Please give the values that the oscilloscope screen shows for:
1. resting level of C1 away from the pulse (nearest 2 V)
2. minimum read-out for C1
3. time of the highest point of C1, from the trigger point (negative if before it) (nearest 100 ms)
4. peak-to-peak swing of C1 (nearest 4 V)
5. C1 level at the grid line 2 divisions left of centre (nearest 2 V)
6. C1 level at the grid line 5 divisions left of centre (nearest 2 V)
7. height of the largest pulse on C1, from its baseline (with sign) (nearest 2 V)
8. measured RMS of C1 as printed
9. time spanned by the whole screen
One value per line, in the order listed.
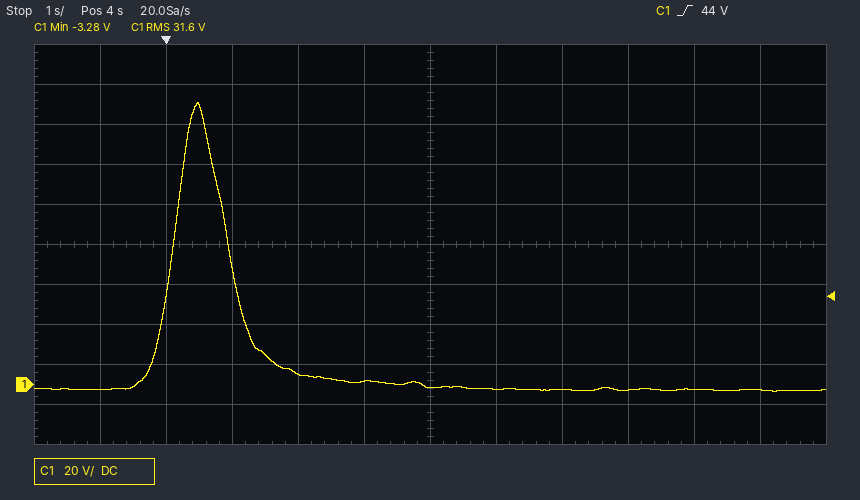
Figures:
-2 V
-3.28 V
+500 ms
144 V
6 V
-2 V
+144 V
31.6 V
12 s
